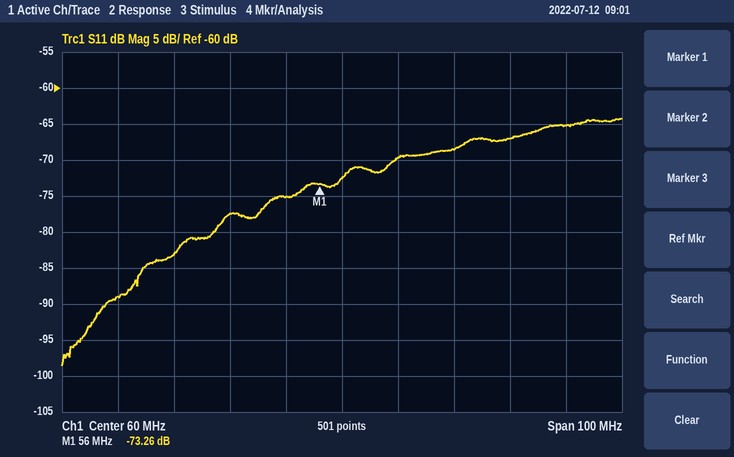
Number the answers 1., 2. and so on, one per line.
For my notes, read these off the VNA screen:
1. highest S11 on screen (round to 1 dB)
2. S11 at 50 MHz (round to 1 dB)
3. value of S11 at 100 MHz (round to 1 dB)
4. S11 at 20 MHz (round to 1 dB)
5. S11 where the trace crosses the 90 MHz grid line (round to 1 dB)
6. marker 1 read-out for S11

1. -64 dB
2. -75 dB
3. -65 dB
4. -89 dB
5. -67 dB
6. -73.26 dB
